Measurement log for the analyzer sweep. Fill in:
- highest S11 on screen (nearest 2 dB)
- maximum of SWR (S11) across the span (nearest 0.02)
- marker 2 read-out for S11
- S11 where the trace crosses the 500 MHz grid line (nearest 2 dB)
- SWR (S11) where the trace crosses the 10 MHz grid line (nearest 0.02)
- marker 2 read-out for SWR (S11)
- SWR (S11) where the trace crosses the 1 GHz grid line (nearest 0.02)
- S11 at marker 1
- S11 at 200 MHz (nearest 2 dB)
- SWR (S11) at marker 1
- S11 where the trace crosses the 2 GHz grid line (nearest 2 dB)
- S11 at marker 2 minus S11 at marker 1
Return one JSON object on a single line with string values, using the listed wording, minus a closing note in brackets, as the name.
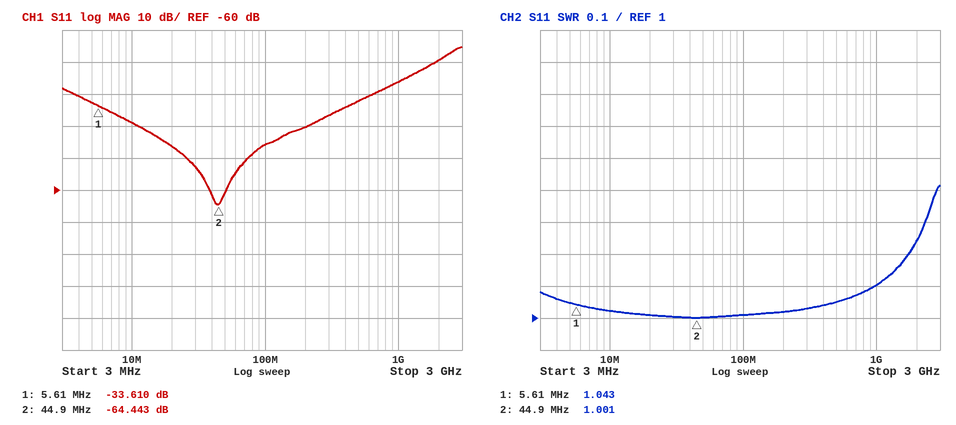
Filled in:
{"highest S11 on screen": "-16 dB", "maximum of SWR (S11) across the span": "1.42", "marker 2 read-out for S11": "-64.443 dB", "S11 where the trace crosses the 500 MHz grid line": "-32 dB", "SWR (S11) where the trace crosses the 10 MHz grid line": "1.02", "marker 2 read-out for SWR": "1.001", "SWR (S11) where the trace crosses the 1 GHz grid line": "1.10", "S11 at marker 1": "-33.610 dB", "S11 at 200 MHz": "-40 dB", "SWR (S11) at marker 1": "1.043", "S11 where the trace crosses the 2 GHz grid line": "-20 dB", "S11 at marker 2 minus S11 at marker 1": "-30.833 dB"}
